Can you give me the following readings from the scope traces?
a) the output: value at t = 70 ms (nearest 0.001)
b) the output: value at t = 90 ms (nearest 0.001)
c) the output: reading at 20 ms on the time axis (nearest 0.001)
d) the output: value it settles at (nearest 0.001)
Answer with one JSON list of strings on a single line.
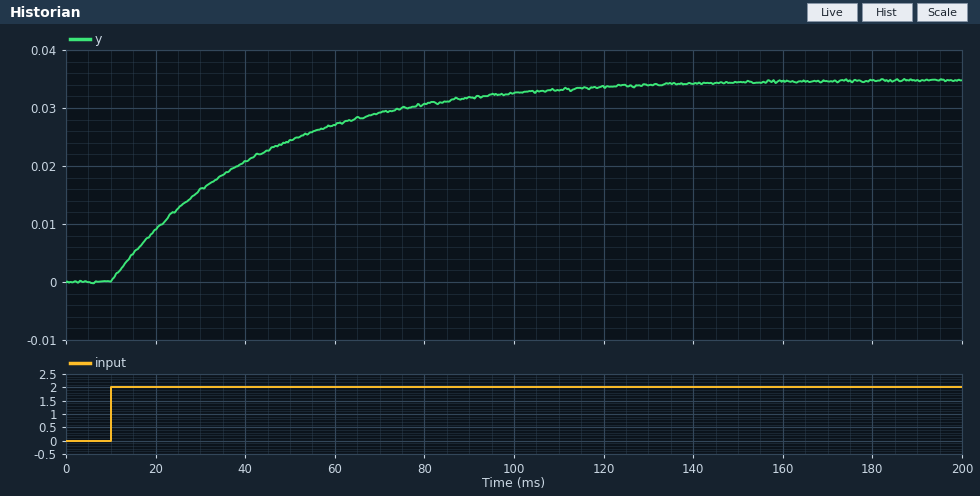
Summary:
["0.029", "0.032", "0.009", "0.035"]
